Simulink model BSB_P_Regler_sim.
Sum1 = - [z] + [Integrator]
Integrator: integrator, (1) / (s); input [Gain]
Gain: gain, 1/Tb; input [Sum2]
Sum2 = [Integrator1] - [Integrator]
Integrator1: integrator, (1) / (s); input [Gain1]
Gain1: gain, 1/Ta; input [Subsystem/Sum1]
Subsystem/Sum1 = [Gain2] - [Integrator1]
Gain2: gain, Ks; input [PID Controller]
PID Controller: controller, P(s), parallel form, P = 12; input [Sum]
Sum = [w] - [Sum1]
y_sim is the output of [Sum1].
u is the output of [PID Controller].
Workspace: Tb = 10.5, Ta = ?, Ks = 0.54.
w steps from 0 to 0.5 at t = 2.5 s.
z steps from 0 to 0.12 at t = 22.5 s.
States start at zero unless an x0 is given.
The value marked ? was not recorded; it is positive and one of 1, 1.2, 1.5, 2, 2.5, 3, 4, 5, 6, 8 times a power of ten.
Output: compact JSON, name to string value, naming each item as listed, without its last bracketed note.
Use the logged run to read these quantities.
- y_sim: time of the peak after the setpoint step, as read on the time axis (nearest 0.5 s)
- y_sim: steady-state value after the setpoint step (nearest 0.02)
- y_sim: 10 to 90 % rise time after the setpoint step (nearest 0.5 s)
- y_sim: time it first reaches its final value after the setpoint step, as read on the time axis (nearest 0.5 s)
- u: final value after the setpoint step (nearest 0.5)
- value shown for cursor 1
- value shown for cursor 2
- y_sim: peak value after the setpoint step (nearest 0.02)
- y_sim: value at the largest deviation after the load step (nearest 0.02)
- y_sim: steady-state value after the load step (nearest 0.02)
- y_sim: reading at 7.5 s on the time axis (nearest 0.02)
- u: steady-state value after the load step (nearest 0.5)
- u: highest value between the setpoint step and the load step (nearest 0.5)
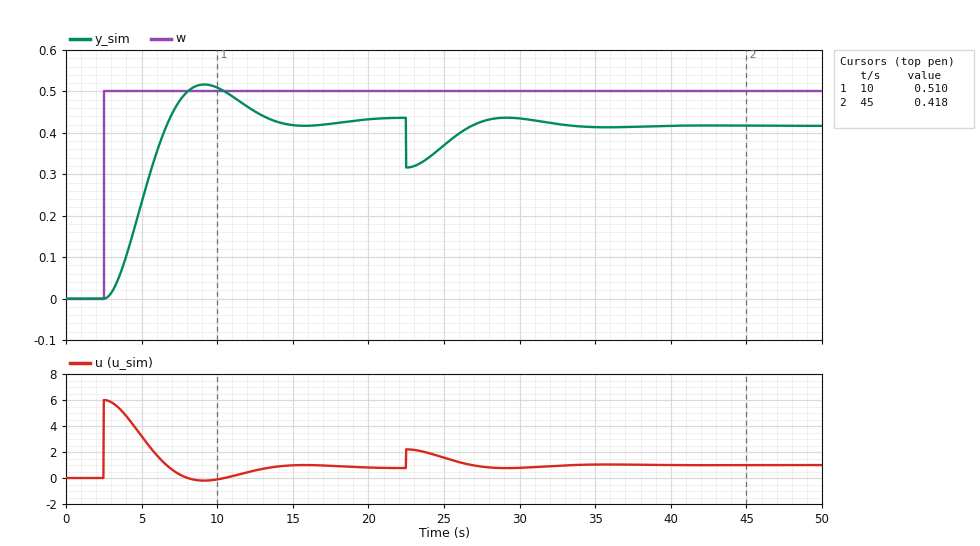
{"y_sim: time of the peak after the setpoint step, as read on the time axis": "9.0 s", "y_sim: steady-state value after the setpoint step": "0.44", "y_sim: 10 to 90 % rise time after the setpoint step": "3.0 s", "y_sim: time it first reaches its final value after the setpoint step, as read on the time axis": "7.0 s", "u: final value after the setpoint step": "1.0", "value shown for cursor 1": "0.510", "value shown for cursor 2": "0.418", "y_sim: peak value after the setpoint step": "0.52", "y_sim: value at the largest deviation after the load step": "0.32", "y_sim: steady-state value after the load step": "0.42", "y_sim: reading at 7.5 s on the time axis": "0.48", "u: steady-state value after the load step": "1.0", "u: highest value between the setpoint step and the load step": "6.0"}
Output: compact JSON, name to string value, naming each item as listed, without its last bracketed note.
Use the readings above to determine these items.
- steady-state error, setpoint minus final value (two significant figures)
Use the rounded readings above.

{"steady-state error, setpoint minus final value": "0.060"}
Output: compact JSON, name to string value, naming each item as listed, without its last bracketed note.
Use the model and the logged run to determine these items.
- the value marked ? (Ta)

{"the value marked ?": "2.5"}
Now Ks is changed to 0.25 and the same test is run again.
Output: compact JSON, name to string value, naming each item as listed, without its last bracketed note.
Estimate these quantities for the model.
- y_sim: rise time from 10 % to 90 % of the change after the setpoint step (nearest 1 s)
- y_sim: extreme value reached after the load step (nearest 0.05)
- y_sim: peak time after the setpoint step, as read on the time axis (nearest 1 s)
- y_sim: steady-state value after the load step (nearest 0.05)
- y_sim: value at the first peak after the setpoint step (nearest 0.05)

{"y_sim: rise time from 10 % to 90 % of the change after the setpoint step": "5 s", "y_sim: extreme value reached after the load step": "0.25", "y_sim: peak time after the setpoint step, as read on the time axis": "13 s", "y_sim: steady-state value after the load step": "0.35", "y_sim: value at the first peak after the setpoint step": "0.40"}
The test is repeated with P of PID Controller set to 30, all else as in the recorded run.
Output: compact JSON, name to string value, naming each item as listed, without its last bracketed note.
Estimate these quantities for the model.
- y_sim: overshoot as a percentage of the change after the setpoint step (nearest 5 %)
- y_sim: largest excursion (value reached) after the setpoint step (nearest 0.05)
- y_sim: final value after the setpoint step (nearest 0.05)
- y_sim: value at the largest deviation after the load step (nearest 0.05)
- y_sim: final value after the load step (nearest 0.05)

{"y_sim: overshoot as a percentage of the change after the setpoint step": "35 %", "y_sim: largest excursion (value reached) after the setpoint step": "0.65", "y_sim: final value after the setpoint step": "0.45", "y_sim: value at the largest deviation after the load step": "0.35", "y_sim: final value after the load step": "0.45"}
